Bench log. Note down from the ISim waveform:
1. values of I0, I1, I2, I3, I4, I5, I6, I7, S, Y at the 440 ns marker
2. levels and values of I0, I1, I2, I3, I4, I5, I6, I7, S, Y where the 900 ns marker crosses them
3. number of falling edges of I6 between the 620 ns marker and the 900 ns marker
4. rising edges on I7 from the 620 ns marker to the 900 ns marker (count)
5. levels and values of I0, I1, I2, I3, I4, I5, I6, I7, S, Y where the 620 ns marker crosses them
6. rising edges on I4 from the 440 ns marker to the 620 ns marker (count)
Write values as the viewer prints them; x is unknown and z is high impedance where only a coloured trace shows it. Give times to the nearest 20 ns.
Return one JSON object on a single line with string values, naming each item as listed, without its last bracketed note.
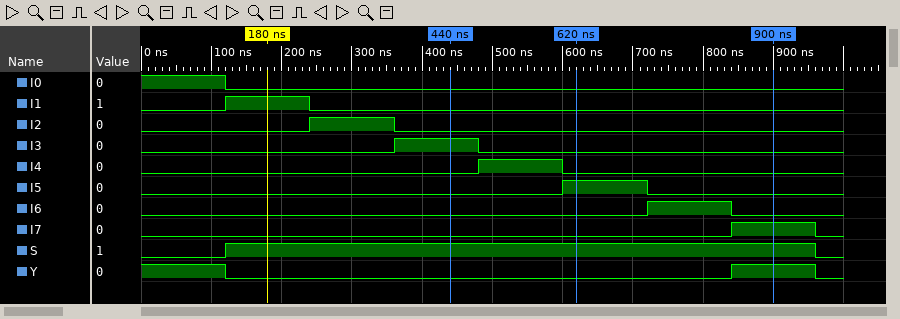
{"values of I0, I1, I2, I3, I4, I5, I6, I7, S, Y at the 440 ns marker": "I0=0, I1=0, I2=0, I3=1, I4=0, I5=0, I6=0, I7=0, S=1, Y=0", "levels and values of I0, I1, I2, I3, I4, I5, I6, I7, S, Y where the 900 ns marker crosses them": "I0=0, I1=0, I2=0, I3=0, I4=0, I5=0, I6=0, I7=1, S=1, Y=1", "number of falling edges of I6 between the 620 ns marker and the 900 ns marker": "1", "rising edges on I7 from the 620 ns marker to the 900 ns marker": "1", "levels and values of I0, I1, I2, I3, I4, I5, I6, I7, S, Y where the 620 ns marker crosses them": "I0=0, I1=0, I2=0, I3=0, I4=0, I5=1, I6=0, I7=0, S=1, Y=0", "rising edges on I4 from the 440 ns marker to the 620 ns marker": "1"}
